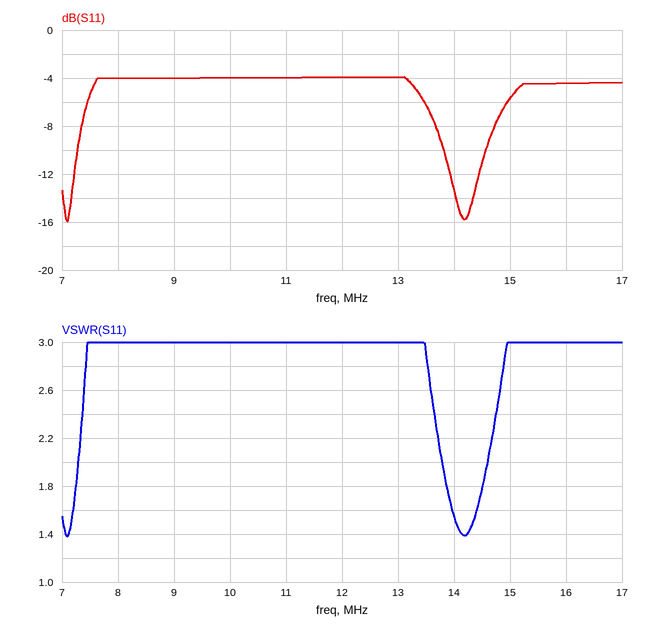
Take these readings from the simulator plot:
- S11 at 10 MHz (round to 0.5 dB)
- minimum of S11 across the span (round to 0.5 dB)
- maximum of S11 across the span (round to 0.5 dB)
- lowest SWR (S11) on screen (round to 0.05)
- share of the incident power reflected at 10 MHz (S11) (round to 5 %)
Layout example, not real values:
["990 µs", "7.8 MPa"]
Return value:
["-4.0 dB", "-16.0 dB", "-4.0 dB", "1.40", "40 %"]
